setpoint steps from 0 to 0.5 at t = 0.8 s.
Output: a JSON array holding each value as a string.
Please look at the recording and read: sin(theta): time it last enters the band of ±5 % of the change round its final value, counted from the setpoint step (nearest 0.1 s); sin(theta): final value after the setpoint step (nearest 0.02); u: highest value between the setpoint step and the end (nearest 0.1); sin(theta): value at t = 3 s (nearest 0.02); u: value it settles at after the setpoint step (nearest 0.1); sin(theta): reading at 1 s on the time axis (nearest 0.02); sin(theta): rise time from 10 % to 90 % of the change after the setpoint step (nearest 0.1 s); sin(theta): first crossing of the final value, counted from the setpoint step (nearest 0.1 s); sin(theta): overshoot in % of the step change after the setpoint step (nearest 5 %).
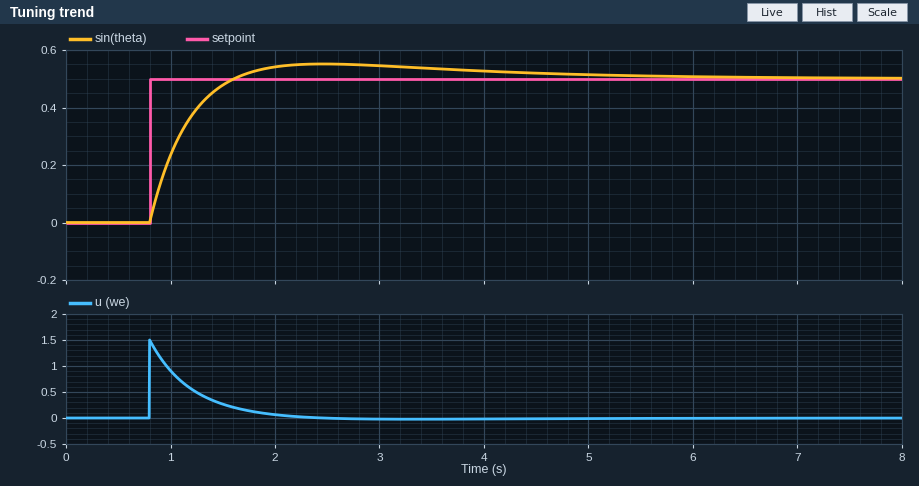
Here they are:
["3.3 s", "0.50", "1.5", "0.54", "0.0", "0.24", "0.6 s", "0.8 s", "10 %"]
